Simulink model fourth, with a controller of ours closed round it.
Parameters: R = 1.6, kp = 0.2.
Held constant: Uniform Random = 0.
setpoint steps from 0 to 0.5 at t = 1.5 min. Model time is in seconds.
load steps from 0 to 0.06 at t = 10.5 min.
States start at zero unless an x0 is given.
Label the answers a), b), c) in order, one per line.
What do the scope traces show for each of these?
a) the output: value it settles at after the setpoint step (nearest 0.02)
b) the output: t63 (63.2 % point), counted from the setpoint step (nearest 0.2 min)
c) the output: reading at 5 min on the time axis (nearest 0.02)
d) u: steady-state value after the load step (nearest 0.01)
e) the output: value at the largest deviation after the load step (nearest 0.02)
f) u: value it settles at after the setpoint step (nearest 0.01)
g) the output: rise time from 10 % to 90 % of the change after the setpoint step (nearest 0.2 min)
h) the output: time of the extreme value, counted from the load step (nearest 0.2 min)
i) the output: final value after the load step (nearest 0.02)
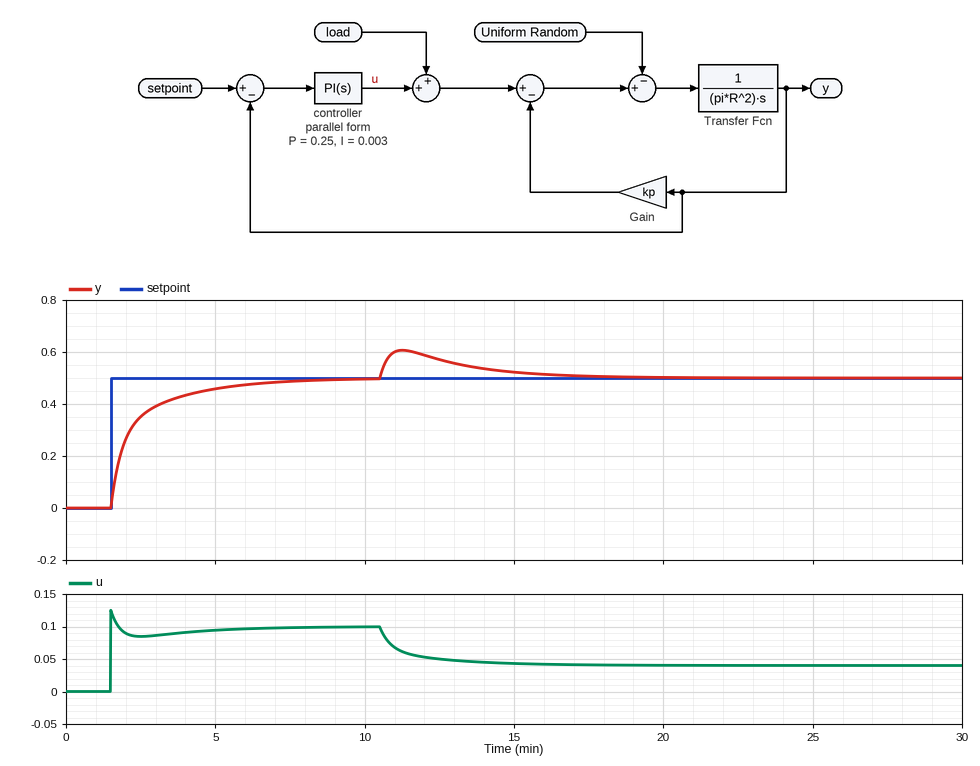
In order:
a) 0.50
b) 0.8 min
c) 0.46
d) 0.04
e) 0.60
f) 0.10
g) 3.0 min
h) 0.8 min
i) 0.50
